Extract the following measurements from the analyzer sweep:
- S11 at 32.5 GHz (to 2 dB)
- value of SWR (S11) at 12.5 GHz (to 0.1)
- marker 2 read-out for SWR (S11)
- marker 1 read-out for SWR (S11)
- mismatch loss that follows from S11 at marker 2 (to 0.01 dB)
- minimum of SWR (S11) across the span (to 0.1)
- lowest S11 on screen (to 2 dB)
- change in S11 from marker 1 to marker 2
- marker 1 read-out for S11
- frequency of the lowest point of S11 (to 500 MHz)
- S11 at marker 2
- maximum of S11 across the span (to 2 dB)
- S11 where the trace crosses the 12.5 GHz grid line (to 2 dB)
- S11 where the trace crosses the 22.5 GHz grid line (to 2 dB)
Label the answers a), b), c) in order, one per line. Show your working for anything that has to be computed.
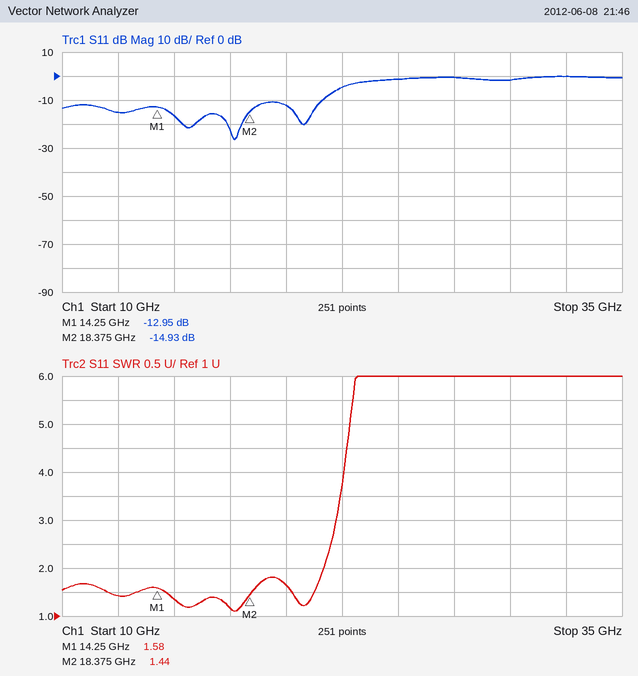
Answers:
a) 0 dB
b) 1.4
c) 1.44
d) 1.58
e) −10 log10(1 − 10^(-14.93/10)) ≈ 0.14 dB
f) 1.1
g) -26 dB
h) -14.93 − (-12.95) = -1.98 dB
i) -12.95 dB
j) 17.5 GHz
k) -14.93 dB
l) 0 dB
m) -16 dB
n) -4 dB
